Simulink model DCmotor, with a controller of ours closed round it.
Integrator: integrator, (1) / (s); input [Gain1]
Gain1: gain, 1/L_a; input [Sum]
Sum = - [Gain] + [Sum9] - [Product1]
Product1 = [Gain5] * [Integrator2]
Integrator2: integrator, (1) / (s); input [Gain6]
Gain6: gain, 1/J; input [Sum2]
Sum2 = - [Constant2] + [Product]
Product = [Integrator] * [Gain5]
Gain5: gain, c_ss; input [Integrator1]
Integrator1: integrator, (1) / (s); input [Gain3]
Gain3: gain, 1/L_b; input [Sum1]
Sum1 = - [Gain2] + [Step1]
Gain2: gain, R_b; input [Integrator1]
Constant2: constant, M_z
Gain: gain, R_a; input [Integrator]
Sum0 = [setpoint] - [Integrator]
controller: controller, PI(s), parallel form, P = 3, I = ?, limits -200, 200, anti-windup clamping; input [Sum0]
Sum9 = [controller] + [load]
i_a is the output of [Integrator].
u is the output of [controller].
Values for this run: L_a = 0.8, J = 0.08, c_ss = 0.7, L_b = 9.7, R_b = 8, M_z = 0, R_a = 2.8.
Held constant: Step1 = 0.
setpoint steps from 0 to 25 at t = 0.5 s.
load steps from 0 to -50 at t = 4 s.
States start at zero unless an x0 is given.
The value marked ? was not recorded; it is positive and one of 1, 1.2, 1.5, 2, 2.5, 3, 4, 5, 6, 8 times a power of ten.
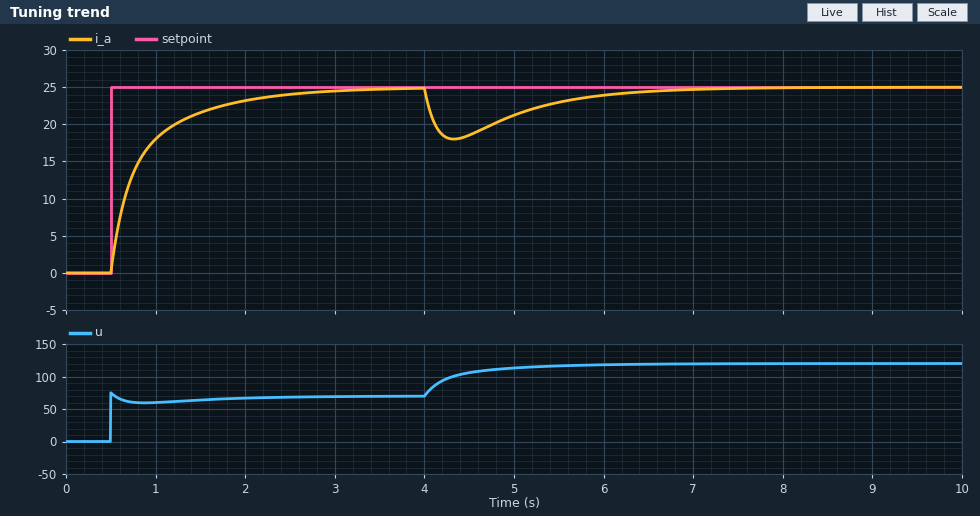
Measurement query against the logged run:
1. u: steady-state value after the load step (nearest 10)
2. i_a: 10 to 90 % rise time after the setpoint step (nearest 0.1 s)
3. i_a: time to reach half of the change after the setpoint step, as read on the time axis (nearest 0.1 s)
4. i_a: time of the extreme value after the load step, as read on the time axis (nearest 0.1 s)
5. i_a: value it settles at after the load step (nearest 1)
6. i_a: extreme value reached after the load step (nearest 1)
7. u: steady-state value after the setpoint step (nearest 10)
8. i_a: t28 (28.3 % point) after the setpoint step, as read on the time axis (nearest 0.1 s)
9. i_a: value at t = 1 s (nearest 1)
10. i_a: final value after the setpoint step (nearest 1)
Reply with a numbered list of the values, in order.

1. 120
2. 1.2 s
3. 0.7 s
4. 4.3 s
5. 25
6. 18
7. 70
8. 0.6 s
9. 18
10. 25
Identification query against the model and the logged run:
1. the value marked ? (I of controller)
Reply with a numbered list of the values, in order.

1. 6
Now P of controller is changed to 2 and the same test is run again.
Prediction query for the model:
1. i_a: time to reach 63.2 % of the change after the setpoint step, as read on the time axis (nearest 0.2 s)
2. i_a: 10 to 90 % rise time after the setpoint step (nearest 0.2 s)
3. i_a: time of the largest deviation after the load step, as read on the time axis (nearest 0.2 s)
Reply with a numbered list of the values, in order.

1. 1.0 s
2. 1.0 s
3. 4.4 s
